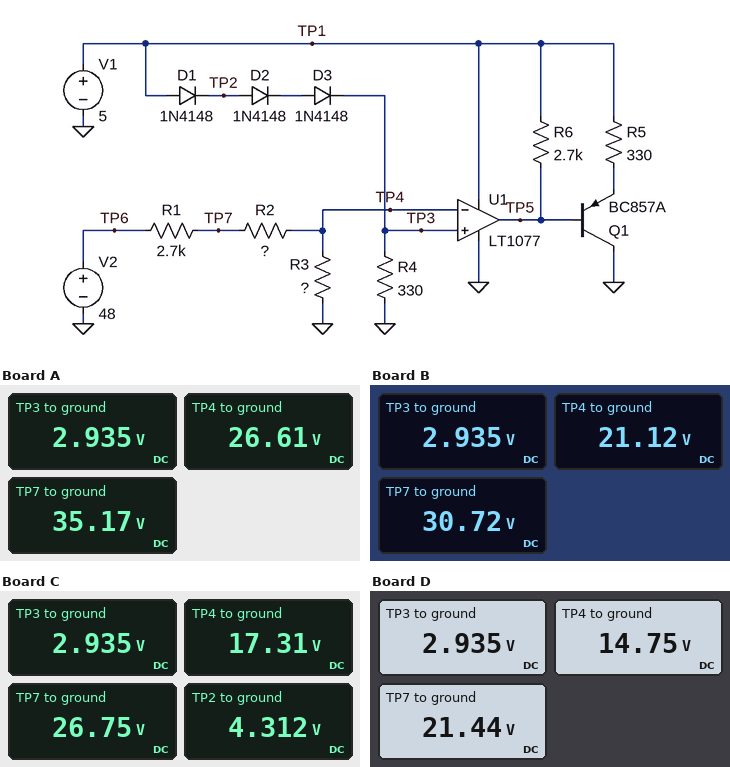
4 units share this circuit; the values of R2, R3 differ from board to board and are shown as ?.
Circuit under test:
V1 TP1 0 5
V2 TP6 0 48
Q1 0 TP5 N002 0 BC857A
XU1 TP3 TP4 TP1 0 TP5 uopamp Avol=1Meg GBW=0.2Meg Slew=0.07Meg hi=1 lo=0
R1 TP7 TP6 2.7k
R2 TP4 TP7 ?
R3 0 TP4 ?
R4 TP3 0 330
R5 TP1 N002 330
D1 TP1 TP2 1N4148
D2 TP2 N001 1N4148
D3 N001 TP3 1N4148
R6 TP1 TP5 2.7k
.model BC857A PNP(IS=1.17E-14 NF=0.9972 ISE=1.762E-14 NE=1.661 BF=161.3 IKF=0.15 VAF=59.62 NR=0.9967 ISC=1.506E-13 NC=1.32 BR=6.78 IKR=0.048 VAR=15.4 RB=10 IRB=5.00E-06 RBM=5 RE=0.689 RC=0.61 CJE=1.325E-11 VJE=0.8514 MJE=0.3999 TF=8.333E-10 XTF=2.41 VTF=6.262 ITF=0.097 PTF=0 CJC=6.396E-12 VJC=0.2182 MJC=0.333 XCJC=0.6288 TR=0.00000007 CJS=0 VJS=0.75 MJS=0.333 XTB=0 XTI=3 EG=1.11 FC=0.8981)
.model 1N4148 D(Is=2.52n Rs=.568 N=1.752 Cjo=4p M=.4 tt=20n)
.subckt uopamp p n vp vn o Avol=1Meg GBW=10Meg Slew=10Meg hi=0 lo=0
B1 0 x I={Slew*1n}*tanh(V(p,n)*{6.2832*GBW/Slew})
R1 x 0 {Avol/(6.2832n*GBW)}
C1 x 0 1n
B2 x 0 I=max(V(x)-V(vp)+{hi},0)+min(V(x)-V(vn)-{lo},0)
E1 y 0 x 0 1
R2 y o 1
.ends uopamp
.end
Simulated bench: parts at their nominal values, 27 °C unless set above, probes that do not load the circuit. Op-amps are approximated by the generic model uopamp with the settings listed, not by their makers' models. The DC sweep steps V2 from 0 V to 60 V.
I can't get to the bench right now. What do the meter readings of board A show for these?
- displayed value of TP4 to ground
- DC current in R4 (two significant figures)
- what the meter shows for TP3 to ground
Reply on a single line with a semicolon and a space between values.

26.61 V; 8.9 mA; 2.935 V
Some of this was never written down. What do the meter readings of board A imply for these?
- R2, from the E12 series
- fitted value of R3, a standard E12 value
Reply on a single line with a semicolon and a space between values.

1.8 kΩ; 5.6 kΩ
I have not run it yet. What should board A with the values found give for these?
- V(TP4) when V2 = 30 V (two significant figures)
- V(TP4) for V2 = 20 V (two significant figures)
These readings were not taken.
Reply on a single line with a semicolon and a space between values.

17 V; 11 V
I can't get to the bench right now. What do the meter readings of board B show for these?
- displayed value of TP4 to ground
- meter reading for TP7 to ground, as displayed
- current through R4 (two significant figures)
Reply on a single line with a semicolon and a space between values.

21.12 V; 30.72 V; 8.9 mA
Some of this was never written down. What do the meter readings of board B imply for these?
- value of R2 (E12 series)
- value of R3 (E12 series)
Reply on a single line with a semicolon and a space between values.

1.5 kΩ; 3.3 kΩ
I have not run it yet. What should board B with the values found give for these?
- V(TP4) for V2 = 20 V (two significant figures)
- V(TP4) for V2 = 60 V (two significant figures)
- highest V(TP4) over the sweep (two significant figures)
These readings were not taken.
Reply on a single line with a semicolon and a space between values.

8.8 V; 26 V; 26 V
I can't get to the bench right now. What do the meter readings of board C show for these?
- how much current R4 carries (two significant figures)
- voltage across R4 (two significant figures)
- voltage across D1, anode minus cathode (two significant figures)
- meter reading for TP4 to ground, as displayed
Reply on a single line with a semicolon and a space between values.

8.9 mA; 2.9 V; 690 mV; 17.31 V
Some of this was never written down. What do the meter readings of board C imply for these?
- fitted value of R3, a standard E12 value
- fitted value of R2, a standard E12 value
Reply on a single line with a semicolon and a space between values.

2.2 kΩ; 1.2 kΩ
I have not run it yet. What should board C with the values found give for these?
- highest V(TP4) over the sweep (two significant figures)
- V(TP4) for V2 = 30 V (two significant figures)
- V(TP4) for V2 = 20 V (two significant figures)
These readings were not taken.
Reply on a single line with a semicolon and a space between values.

22 V; 11 V; 7.2 V
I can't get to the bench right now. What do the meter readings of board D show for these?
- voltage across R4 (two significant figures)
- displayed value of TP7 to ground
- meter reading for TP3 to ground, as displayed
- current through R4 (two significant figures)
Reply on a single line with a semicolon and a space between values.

2.9 V; 21.44 V; 2.935 V; 8.9 mA
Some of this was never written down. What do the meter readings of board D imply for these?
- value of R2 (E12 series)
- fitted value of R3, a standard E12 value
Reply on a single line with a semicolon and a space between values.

680 Ω; 1.5 kΩ
